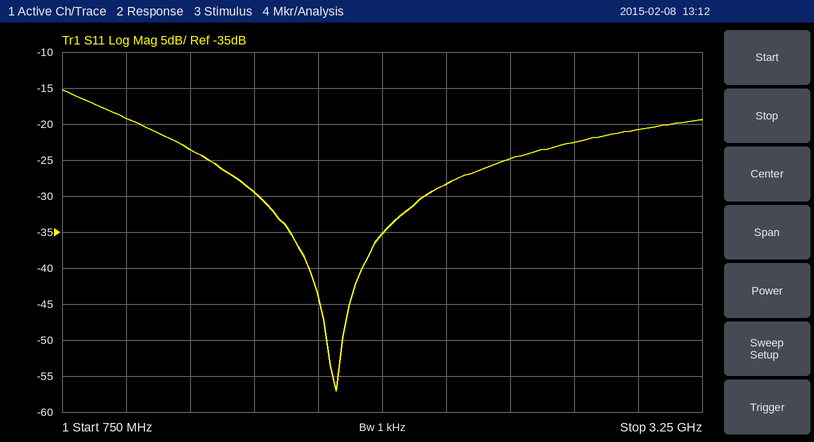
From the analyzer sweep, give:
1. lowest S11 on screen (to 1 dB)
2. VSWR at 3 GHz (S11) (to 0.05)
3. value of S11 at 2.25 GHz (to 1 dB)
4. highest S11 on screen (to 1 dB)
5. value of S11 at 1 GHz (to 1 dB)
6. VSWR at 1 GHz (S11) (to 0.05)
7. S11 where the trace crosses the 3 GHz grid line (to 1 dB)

-57 dB
1.20
-28 dB
-15 dB
-19 dB
1.25
-21 dB
